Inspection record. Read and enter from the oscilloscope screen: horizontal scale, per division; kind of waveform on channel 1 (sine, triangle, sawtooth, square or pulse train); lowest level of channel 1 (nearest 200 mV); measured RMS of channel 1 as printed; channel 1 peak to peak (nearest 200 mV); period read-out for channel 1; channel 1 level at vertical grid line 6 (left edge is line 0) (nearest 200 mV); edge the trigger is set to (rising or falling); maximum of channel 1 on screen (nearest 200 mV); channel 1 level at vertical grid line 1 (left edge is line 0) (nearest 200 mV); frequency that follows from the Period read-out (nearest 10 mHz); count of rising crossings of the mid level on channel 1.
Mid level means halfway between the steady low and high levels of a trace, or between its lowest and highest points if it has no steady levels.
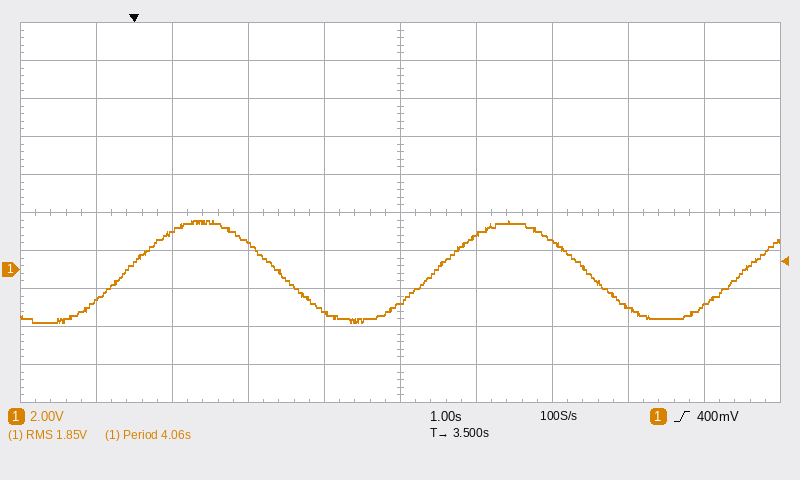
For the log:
1 s
sine
-2.8 V
1.85 V
5.4 V
4.06 s
1.8 V
rising
2.6 V
-1.6 V
250 mHz
3
